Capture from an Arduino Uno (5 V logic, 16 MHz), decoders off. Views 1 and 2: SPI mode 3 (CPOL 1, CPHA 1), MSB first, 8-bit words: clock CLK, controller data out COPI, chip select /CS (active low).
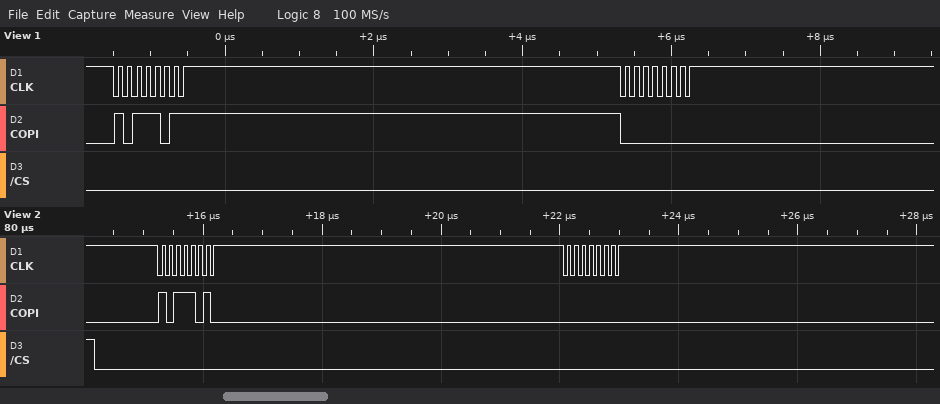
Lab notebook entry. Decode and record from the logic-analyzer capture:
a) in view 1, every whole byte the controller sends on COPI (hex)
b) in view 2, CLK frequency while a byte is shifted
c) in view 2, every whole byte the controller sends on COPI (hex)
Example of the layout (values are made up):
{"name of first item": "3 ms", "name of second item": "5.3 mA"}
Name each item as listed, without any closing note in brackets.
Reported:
{"in view 1, every whole byte the controller sends on COPI": "BB 00", "in view 2, CLK frequency while a byte is shifted": "8 MHz", "in view 2, every whole byte the controller sends on COPI": "BA 00"}
